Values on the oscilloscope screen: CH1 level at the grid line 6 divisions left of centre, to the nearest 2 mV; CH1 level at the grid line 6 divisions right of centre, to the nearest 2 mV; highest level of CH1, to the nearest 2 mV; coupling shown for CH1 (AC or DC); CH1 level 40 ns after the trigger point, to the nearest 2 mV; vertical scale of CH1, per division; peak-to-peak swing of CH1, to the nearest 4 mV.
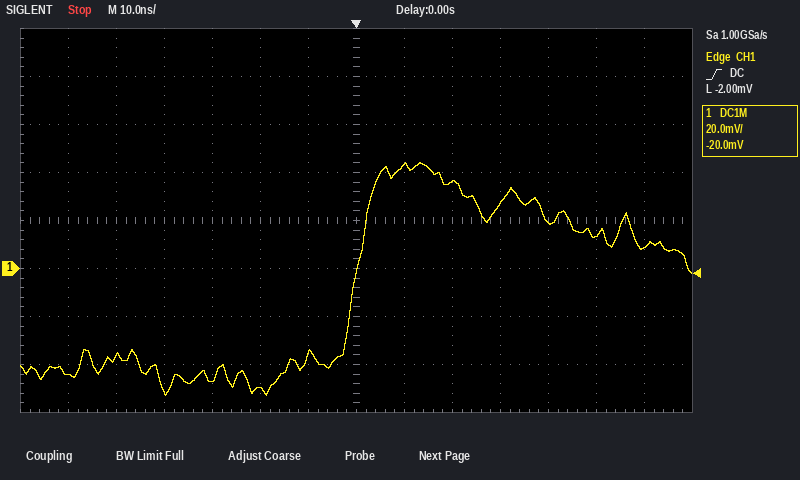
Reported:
-44 mV
8 mV
44 mV
DC
20 mV
20 mV
96 mV
